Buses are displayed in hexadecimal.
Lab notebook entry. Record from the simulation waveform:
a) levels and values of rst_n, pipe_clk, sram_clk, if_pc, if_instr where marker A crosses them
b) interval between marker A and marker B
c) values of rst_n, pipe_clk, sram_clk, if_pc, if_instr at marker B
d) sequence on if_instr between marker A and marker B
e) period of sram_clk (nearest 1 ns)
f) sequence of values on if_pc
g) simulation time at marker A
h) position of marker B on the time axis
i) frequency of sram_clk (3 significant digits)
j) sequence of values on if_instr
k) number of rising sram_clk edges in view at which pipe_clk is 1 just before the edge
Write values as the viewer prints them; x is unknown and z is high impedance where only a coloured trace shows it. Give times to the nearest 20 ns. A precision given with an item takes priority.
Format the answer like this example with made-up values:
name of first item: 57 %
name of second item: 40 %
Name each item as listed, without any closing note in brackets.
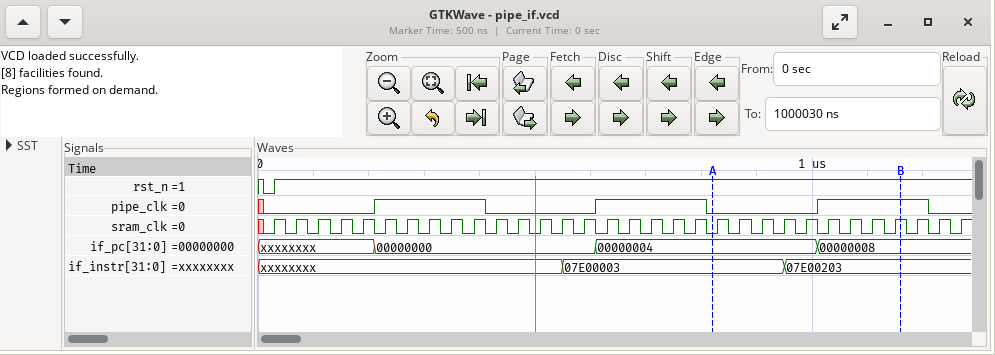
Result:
levels and values of rst_n, pipe_clk, sram_clk, if_pc, if_instr where marker A crosses them: rst_n=1, pipe_clk=0, sram_clk=0, if_pc=00000004, if_instr=07E00003
interval between marker A and marker B: 340 ns
values of rst_n, pipe_clk, sram_clk, if_pc, if_instr at marker B: rst_n=1, pipe_clk=1, sram_clk=1, if_pc=00000008, if_instr=07E00203
sequence on if_instr between marker A and marker B: 07E00003, 07E00203
period of sram_clk: 40 ns
sequence of values on if_pc: xxxxxxxx, 00000000, 00000004, 00000008
simulation time at marker A: 820 ns
position of marker B on the time axis: 1160 ns
frequency of sram_clk: 25.0 MHz
sequence of values on if_instr: xxxxxxxx, 07E00003, 07E00203
number of rising sram_clk edges in view at which pipe_clk is 1 just before the edge: 15
